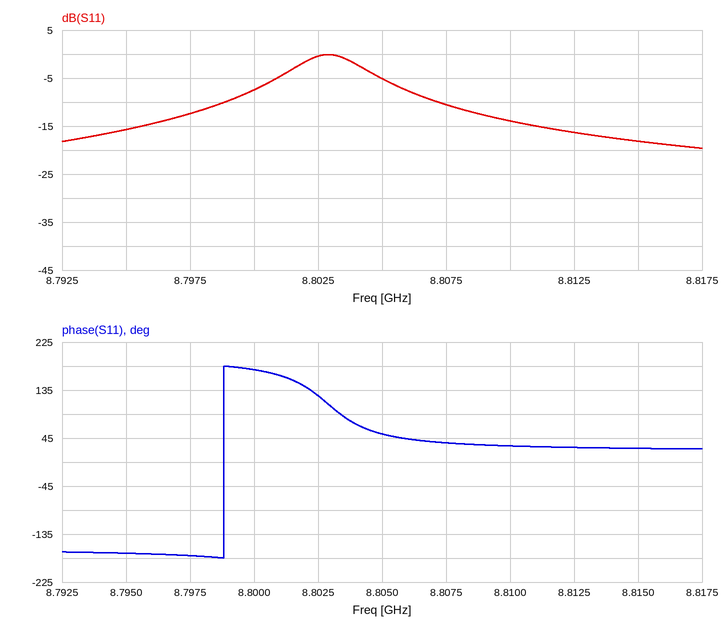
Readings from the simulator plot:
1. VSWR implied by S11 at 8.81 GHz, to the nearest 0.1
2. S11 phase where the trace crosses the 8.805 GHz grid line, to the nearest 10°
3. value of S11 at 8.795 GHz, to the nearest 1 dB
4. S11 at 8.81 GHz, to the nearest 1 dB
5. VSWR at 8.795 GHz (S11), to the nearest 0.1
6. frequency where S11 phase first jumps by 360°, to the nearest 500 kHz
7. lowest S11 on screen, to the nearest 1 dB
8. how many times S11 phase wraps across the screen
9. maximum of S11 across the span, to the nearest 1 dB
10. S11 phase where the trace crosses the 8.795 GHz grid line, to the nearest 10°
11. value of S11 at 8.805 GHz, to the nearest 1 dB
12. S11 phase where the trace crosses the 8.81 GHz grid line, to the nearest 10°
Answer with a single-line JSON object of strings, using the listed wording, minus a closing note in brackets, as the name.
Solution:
{"VSWR implied by S11 at 8.81 GHz, to the nearest 0.1": "1.5", "S11 phase where the trace crosses the 8.805 GHz grid line, to the nearest 10°": "50°", "value of S11 at 8.795 GHz, to the nearest 1 dB": "-16 dB", "S11 at 8.81 GHz, to the nearest 1 dB": "-14 dB", "VSWR at 8.795 GHz (S11), to the nearest 0.1": "1.4", "frequency where S11 phase first jumps by 360°, to the nearest 500 kHz": "8.7990 GHz", "lowest S11 on screen, to the nearest 1 dB": "-20 dB", "how many times S11 phase wraps across the screen": "1", "maximum of S11 across the span, to the nearest 1 dB": "0 dB", "S11 phase where the trace crosses the 8.795 GHz grid line, to the nearest 10°": "-170°", "value of S11 at 8.805 GHz, to the nearest 1 dB": "-5 dB", "S11 phase where the trace crosses the 8.81 GHz grid line, to the nearest 10°": "30°"}
